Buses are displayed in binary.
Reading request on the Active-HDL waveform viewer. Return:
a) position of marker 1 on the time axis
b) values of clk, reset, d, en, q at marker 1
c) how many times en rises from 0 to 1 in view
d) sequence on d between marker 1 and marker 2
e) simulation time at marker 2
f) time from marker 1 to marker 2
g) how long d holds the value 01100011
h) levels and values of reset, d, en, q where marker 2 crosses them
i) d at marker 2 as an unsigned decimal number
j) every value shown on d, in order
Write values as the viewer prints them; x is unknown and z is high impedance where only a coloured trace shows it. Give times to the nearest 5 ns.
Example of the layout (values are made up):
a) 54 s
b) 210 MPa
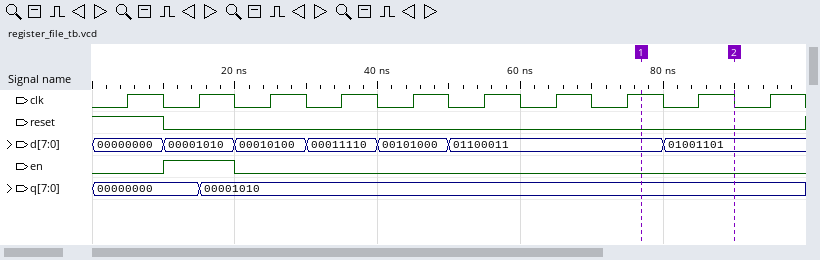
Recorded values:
a) 75 ns
b) clk=1, reset=0, d=01100011, en=0, q=00001010
c) 1
d) 01100011, 01001101
e) 90 ns
f) 15 ns
g) 30 ns
h) reset=0, d=01001101, en=0, q=00001010
i) 77
j) 00000000, 00001010, 00010100, 00011110, 00101000, 01100011, 01001101
